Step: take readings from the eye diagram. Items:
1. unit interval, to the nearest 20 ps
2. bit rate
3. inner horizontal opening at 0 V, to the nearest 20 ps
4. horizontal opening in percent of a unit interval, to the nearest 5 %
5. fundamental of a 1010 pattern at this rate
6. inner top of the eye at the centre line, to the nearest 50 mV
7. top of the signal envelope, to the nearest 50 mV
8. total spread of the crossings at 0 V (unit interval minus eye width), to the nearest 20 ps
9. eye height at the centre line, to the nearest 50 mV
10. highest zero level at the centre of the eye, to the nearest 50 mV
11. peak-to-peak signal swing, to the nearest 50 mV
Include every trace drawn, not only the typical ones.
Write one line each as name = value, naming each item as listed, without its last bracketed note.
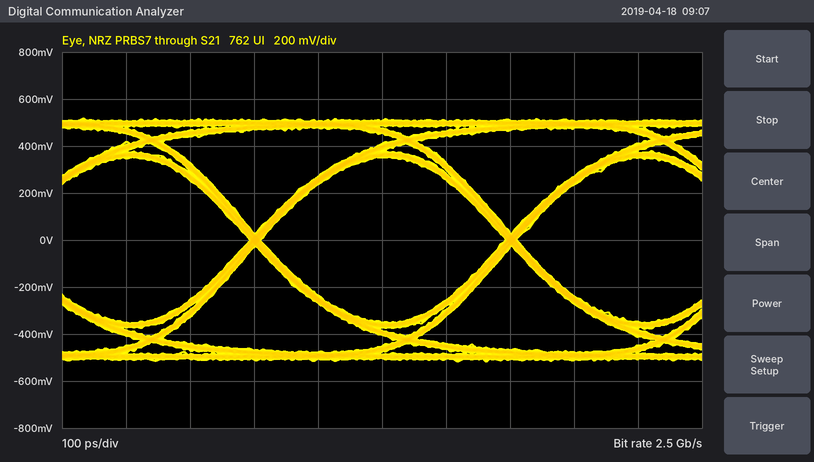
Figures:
unit interval, to the nearest 20 ps = 400 ps
bit rate = 2.5 Gb/s
inner horizontal opening at 0 V, to the nearest 20 ps = 380 ps
horizontal opening in percent of a unit interval, to the nearest 5 % = 95 %
fundamental of a 1010 pattern at this rate = 1.25 GHz
inner top of the eye at the centre line, to the nearest 50 mV = 350 mV
top of the signal envelope, to the nearest 50 mV = 500 mV
total spread of the crossings at 0 V (unit interval minus eye width), to the nearest 20 ps = 20 ps
eye height at the centre line, to the nearest 50 mV = 700 mV
highest zero level at the centre of the eye, to the nearest 50 mV = -350 mV
peak-to-peak signal swing, to the nearest 50 mV = 1.05 V
